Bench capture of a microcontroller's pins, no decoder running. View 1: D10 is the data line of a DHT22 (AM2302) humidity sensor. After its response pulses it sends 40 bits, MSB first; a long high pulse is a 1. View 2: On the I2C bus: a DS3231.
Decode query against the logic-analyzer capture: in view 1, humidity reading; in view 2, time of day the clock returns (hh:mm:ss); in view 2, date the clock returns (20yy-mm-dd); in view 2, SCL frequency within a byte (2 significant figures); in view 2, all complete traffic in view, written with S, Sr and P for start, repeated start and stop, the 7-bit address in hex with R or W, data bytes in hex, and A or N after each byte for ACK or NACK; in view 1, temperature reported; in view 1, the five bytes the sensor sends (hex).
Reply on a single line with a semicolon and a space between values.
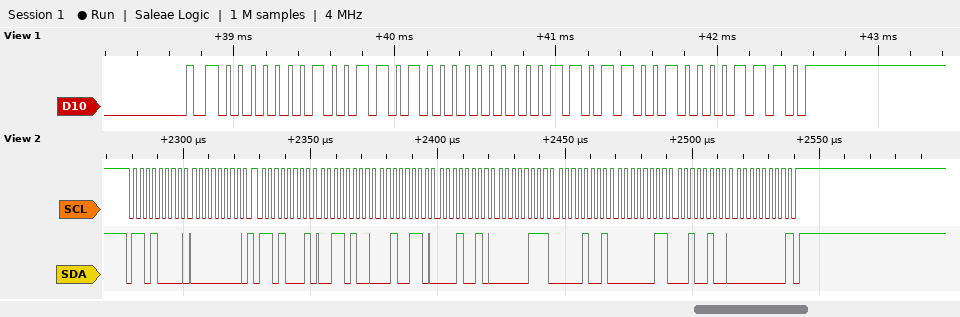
30.8 %; 12:26:34; 2024-03-09; 400 kHz; S 68W A 00 A Sr 68R A 34 A 26 A 12 A 07 A 09 A 03 A 24 A 00 N P; 21.7 °C; 01 34 00 D9 0E
